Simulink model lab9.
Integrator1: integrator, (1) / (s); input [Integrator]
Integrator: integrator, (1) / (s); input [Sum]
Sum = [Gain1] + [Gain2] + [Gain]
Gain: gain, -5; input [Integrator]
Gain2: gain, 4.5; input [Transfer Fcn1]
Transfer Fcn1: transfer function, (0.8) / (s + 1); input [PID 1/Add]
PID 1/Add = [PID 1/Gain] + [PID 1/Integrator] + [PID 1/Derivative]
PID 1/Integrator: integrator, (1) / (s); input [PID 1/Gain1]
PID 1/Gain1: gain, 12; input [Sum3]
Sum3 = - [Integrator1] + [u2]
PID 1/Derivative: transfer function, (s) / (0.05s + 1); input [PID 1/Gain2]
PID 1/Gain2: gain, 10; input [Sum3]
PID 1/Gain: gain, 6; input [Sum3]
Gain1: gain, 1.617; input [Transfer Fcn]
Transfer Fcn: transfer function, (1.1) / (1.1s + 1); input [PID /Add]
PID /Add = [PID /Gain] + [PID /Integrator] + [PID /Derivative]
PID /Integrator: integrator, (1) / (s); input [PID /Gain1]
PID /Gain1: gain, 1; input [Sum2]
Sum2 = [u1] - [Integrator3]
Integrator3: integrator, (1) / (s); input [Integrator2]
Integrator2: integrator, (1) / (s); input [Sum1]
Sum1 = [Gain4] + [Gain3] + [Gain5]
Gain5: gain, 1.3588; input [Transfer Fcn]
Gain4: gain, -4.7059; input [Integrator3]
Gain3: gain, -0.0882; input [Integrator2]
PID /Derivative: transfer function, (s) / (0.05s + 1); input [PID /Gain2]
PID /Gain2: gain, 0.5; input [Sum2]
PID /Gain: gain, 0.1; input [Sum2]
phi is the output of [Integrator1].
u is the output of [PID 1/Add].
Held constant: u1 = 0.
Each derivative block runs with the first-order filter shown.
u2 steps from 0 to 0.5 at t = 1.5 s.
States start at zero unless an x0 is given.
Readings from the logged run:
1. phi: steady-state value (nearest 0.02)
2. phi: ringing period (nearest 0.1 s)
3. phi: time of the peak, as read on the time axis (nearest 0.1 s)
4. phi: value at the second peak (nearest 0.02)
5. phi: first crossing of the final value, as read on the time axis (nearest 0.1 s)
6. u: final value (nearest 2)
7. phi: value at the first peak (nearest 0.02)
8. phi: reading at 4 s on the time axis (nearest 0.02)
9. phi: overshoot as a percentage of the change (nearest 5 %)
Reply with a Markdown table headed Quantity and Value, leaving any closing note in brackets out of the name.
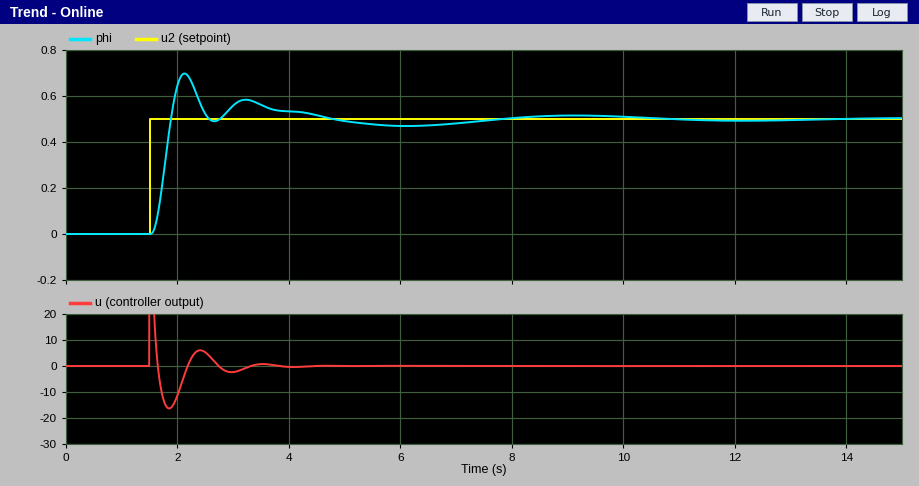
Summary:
| Quantity | Value |
|---|---|
| phi: steady-state value | 0.50 |
| phi: ringing period | 1.1 s |
| phi: time of the peak, as read on the time axis | 2.1 s |
| phi: value at the second peak | 0.58 |
| phi: first crossing of the final value, as read on the time axis | 1.9 s |
| u: final value | 0 |
| phi: value at the first peak | 0.70 |
| phi: reading at 4 s on the time axis | 0.54 |
| phi: overshoot as a percentage of the change | 40 % |
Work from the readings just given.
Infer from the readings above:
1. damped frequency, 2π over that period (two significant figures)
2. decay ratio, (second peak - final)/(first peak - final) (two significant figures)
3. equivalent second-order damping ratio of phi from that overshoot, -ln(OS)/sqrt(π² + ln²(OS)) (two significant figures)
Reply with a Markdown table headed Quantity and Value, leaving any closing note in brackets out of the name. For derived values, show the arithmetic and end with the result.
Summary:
| Quantity | Value |
|---|---|
| damped frequency, 2π over that period | 2π / 1.1 = 5.7 rad/s |
| decay ratio, (second peak - final)/(first peak - final) | (0.58 - 0.5) / (0.7 - 0.5) = 0.40 |
| equivalent second-order damping ratio of phi from that overshoot, -ln(OS)/sqrt(π² + ln²(OS)) | ln(0.4) = -0.916; 0.916 / sqrt(9.870 + 0.840) = 0.28 |
